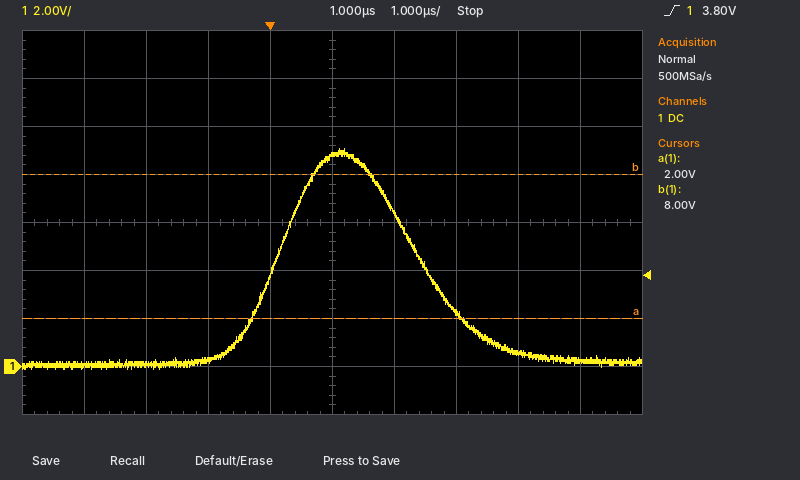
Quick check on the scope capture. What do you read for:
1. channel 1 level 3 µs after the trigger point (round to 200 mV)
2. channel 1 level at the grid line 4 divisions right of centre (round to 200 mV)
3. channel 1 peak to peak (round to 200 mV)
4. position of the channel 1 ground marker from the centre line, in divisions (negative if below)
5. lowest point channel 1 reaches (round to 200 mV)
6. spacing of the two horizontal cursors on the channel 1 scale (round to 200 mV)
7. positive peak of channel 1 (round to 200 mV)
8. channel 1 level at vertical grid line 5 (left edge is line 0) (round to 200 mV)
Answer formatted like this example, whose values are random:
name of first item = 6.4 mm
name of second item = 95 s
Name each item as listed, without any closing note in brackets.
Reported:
channel 1 level 3 µs after the trigger point = 2.2 V
channel 1 level at the grid line 4 divisions right of centre = 200 mV
channel 1 peak to peak = 9.2 V
position of the channel 1 ground marker from the centre line, in divisions = -3.0 div
lowest point channel 1 reaches = -200 mV
spacing of the two horizontal cursors on the channel 1 scale = 6.0 V
positive peak of channel 1 = 9.0 V
channel 1 level at vertical grid line 5 (left edge is line 0) = 8.8 V
